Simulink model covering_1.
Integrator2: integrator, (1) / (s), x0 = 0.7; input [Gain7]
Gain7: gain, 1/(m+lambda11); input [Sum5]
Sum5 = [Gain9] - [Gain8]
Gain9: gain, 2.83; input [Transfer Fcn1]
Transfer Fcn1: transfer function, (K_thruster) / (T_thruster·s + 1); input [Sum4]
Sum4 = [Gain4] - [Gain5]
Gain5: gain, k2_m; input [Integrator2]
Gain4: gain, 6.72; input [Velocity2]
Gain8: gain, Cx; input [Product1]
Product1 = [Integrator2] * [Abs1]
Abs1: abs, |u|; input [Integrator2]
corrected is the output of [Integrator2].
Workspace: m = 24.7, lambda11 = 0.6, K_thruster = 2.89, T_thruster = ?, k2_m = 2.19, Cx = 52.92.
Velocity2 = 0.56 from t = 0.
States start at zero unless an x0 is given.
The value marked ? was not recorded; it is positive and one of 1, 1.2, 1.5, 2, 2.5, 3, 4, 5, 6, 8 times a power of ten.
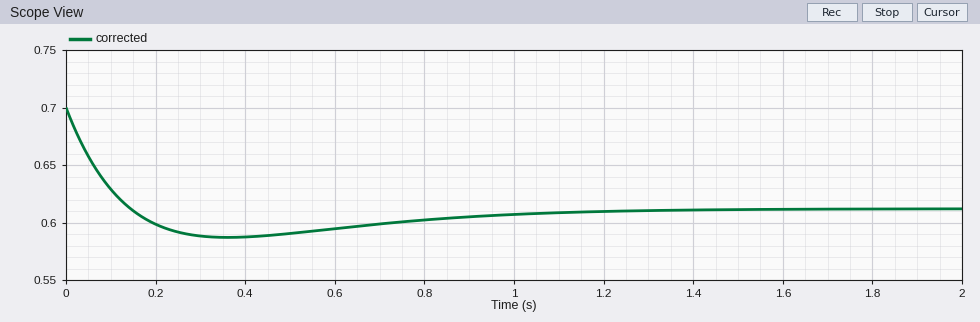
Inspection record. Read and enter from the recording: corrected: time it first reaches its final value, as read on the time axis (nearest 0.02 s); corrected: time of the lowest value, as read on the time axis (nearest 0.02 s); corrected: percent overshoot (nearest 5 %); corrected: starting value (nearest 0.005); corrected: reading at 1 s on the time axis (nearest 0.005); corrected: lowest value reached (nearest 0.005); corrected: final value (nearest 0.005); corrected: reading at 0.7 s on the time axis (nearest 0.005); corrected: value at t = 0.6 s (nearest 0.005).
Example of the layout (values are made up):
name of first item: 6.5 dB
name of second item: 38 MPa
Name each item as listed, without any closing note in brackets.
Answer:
corrected: time it first reaches its final value, as read on the time axis: 0.14 s
corrected: time of the lowest value, as read on the time axis: 0.36 s
corrected: percent overshoot: 30 %
corrected: starting value: 0.700
corrected: reading at 1 s on the time axis: 0.605
corrected: lowest value reached: 0.585
corrected: final value: 0.610
corrected: reading at 0.7 s on the time axis: 0.600
corrected: value at t = 0.6 s: 0.595
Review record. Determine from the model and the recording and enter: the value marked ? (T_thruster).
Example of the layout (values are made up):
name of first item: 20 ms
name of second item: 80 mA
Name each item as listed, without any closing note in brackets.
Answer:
the value marked ?: 0.15
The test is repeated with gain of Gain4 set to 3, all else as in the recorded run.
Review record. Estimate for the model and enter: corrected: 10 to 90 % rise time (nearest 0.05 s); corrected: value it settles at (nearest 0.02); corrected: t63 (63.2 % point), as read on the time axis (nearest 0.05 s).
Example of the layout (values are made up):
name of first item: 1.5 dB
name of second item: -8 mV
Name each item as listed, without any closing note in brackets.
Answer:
corrected: 10 to 90 % rise time: 0.75 s
corrected: value it settles at: 0.36
corrected: t63 (63.2 % point), as read on the time axis: 0.35 s
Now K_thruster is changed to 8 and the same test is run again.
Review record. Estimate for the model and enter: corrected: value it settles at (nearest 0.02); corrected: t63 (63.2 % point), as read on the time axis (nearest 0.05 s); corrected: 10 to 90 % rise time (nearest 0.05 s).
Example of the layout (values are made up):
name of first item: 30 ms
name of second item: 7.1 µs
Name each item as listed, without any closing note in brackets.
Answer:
corrected: value it settles at: 0.88
corrected: t63 (63.2 % point), as read on the time axis: 0.45 s
corrected: 10 to 90 % rise time: 0.40 s
